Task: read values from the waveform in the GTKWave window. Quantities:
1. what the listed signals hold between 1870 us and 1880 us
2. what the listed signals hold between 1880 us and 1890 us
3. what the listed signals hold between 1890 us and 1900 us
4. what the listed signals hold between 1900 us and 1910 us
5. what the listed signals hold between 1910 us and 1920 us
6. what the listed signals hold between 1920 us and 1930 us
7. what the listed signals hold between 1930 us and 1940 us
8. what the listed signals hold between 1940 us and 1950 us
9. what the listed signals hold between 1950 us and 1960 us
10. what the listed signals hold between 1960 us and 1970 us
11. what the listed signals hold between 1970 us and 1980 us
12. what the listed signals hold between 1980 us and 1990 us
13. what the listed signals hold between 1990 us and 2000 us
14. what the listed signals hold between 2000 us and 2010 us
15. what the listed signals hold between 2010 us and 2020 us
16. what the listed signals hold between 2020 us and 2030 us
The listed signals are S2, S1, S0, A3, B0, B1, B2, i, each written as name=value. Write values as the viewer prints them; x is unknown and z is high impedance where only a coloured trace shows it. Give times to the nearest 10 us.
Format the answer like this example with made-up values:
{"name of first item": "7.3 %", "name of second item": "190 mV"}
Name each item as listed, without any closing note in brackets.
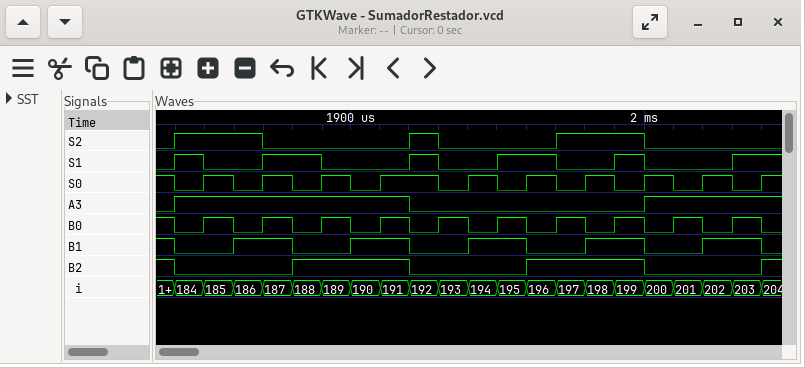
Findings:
{"what the listed signals hold between 1870 us and 1880 us": "S2=0, S1=1, S0=1, A3=1, B0=1, B1=1, B2=0, i=187", "what the listed signals hold between 1880 us and 1890 us": "S2=0, S1=1, S0=0, A3=1, B0=0, B1=0, B2=1, i=188", "what the listed signals hold between 1890 us and 1900 us": "S2=0, S1=0, S0=1, A3=1, B0=1, B1=0, B2=1, i=189", "what the listed signals hold between 1900 us and 1910 us": "S2=0, S1=0, S0=0, A3=1, B0=0, B1=1, B2=1, i=190", "what the listed signals hold between 1910 us and 1920 us": "S2=0, S1=0, S0=1, A3=1, B0=1, B1=1, B2=1, i=191", "what the listed signals hold between 1920 us and 1930 us": "S2=1, S1=1, S0=1, A3=0, B0=0, B1=0, B2=0, i=192", "what the listed signals hold between 1930 us and 1940 us": "S2=0, S1=0, S0=0, A3=0, B0=1, B1=0, B2=0, i=193", "what the listed signals hold between 1940 us and 1950 us": "S2=0, S1=0, S0=1, A3=0, B0=0, B1=1, B2=0, i=194", "what the listed signals hold between 1950 us and 1960 us": "S2=0, S1=1, S0=0, A3=0, B0=1, B1=1, B2=0, i=195", "what the listed signals hold between 1960 us and 1970 us": "S2=0, S1=1, S0=1, A3=0, B0=0, B1=0, B2=1, i=196", "what the listed signals hold between 1970 us and 1980 us": "S2=1, S1=0, S0=0, A3=0, B0=1, B1=0, B2=1, i=197", "what the listed signals hold between 1980 us and 1990 us": "S2=1, S1=0, S0=1, A3=0, B0=0, B1=1, B2=1, i=198", "what the listed signals hold between 1990 us and 2000 us": "S2=1, S1=1, S0=0, A3=0, B0=1, B1=1, B2=1, i=199", "what the listed signals hold between 2000 us and 2010 us": "S2=0, S1=0, S0=1, A3=1, B0=0, B1=0, B2=0, i=200", "what the listed signals hold between 2010 us and 2020 us": "S2=0, S1=0, S0=0, A3=1, B0=1, B1=0, B2=0, i=201", "what the listed signals hold between 2020 us and 2030 us": "S2=0, S1=0, S0=1, A3=1, B0=0, B1=1, B2=0, i=202"}
